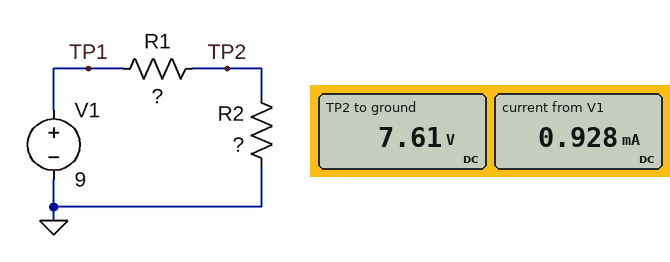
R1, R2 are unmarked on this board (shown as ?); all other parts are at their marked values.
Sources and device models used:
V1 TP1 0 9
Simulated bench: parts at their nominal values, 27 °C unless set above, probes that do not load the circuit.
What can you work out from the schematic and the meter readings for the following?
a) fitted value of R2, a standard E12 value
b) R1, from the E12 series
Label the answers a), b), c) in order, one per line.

a) 8.2 kΩ
b) 1.5 kΩ
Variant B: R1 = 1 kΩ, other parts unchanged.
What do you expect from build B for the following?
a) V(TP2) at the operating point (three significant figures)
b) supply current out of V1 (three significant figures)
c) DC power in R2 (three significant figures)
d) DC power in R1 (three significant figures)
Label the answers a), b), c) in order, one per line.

a) 8.02 V
b) 978 µA
c) 7.85 mW
d) 957 µW
